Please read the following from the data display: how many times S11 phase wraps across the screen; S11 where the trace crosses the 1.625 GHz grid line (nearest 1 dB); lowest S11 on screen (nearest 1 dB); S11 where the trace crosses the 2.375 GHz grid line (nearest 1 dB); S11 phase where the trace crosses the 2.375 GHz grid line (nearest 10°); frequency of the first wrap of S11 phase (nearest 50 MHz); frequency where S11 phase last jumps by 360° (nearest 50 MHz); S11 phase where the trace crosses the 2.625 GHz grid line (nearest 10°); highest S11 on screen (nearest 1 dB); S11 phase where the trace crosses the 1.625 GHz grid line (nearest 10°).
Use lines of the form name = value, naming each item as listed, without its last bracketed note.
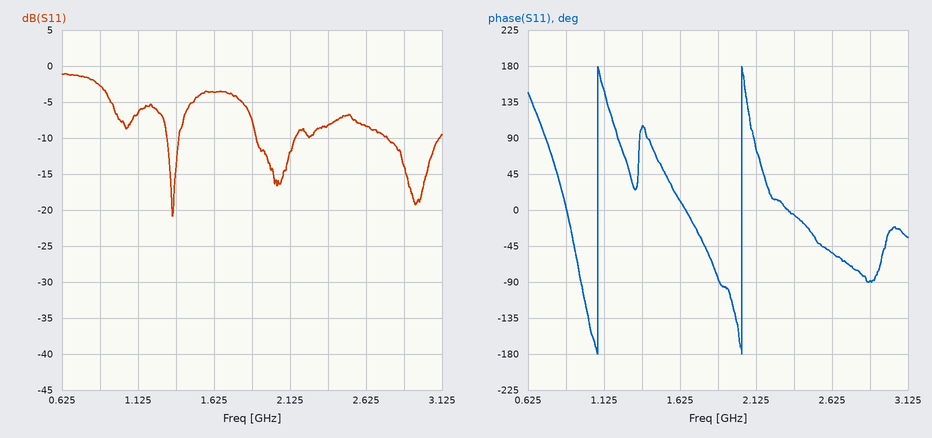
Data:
how many times S11 phase wraps across the screen = 2
S11 where the trace crosses the 1.625 GHz grid line = -4 dB
lowest S11 on screen = -21 dB
S11 where the trace crosses the 2.375 GHz grid line = -8 dB
S11 phase where the trace crosses the 2.375 GHz grid line = -10°
frequency of the first wrap of S11 phase = 1.10 GHz
frequency where S11 phase last jumps by 360° = 2.05 GHz
S11 phase where the trace crosses the 2.625 GHz grid line = -50°
highest S11 on screen = -1 dB
S11 phase where the trace crosses the 1.625 GHz grid line = 10°
